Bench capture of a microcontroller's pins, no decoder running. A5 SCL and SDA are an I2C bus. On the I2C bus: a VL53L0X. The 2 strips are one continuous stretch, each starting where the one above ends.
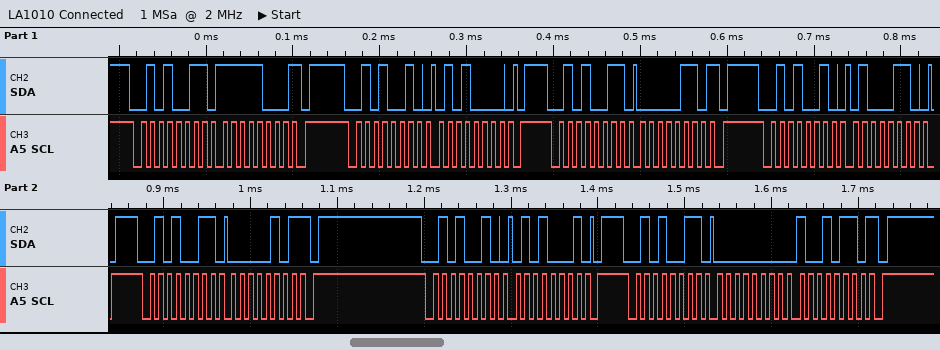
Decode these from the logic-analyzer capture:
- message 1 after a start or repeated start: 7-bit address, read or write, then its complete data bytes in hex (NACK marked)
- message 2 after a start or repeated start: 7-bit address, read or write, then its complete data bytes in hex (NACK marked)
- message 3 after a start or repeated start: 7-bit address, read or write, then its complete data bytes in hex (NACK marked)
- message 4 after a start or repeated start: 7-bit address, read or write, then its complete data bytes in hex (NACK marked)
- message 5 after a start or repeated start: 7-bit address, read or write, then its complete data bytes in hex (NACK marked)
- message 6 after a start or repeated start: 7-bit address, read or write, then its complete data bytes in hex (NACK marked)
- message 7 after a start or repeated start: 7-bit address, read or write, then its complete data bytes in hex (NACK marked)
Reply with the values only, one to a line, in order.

0x29 read: F8 NACK
0x29 write: 50
0x29 read: 06 NACK
0x29 write: 46
0x29 read: 05 NACK
0x29 write: 51
0x29 read: 00 96 NACK
